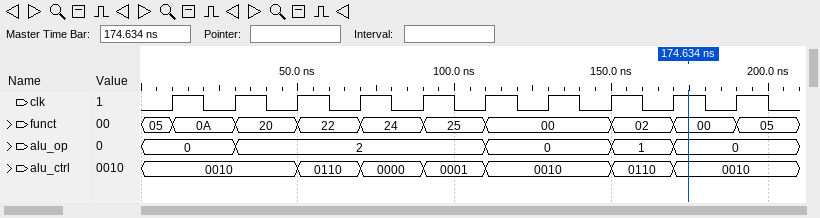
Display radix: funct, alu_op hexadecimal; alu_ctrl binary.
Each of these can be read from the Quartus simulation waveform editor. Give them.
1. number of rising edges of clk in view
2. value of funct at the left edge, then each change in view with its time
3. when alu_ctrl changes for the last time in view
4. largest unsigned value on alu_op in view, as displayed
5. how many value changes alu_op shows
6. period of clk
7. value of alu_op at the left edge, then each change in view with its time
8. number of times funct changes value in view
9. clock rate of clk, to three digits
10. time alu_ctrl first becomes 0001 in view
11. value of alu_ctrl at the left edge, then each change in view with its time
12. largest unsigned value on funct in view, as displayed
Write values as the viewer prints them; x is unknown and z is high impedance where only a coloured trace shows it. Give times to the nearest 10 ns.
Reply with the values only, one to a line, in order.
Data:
10
05, 0A at 10 ns, 20 at 30 ns, 22 at 50 ns, 24 at 70 ns, 25 at 90 ns, 00 at 110 ns, 02 at 150 ns, 00 at 170 ns, 05 at 190 ns
170 ns
2
4
20 ns
0, 2 at 30 ns, 0 at 110 ns, 1 at 150 ns, 0 at 170 ns
9
50.0 MHz
90 ns
0010, 0110 at 50 ns, 0000 at 70 ns, 0001 at 90 ns, 0010 at 110 ns, 0110 at 150 ns, 0010 at 170 ns
25
